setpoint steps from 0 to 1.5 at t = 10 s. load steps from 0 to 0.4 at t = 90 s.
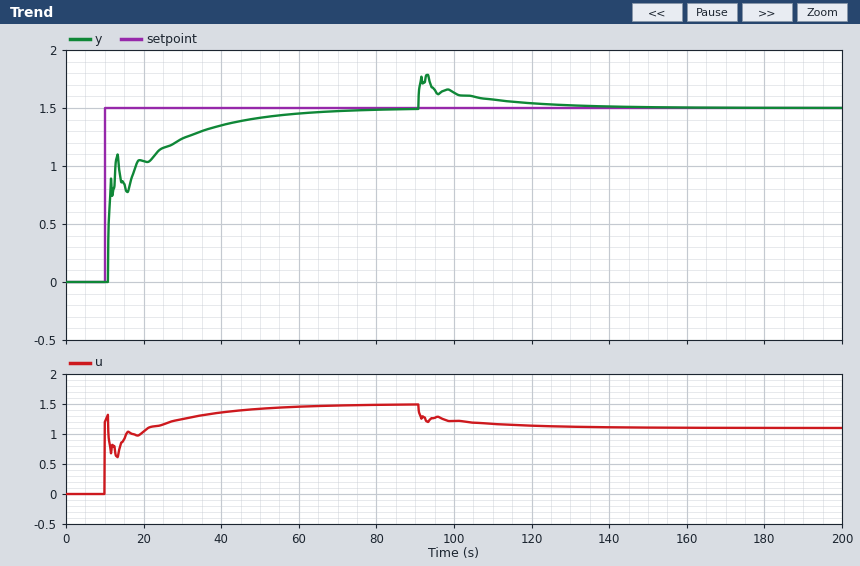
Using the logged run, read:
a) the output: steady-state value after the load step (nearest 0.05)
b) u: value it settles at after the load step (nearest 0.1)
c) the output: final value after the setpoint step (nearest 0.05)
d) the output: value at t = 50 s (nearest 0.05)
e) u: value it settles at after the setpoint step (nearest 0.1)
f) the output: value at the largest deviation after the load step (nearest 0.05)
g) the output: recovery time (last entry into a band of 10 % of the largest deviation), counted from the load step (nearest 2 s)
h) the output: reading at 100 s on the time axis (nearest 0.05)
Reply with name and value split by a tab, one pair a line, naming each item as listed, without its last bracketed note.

the output: steady-state value after the load step	1.50
u: value it settles at after the load step	1.1
the output: final value after the setpoint step	1.50
the output: value at t = 50 s	1.40
u: value it settles at after the setpoint step	1.5
the output: value at the largest deviation after the load step	1.80
the output: recovery time (last entry into a band of 10 % of the largest deviation), counted from the load step	36 s
the output: reading at 100 s on the time axis	1.65
